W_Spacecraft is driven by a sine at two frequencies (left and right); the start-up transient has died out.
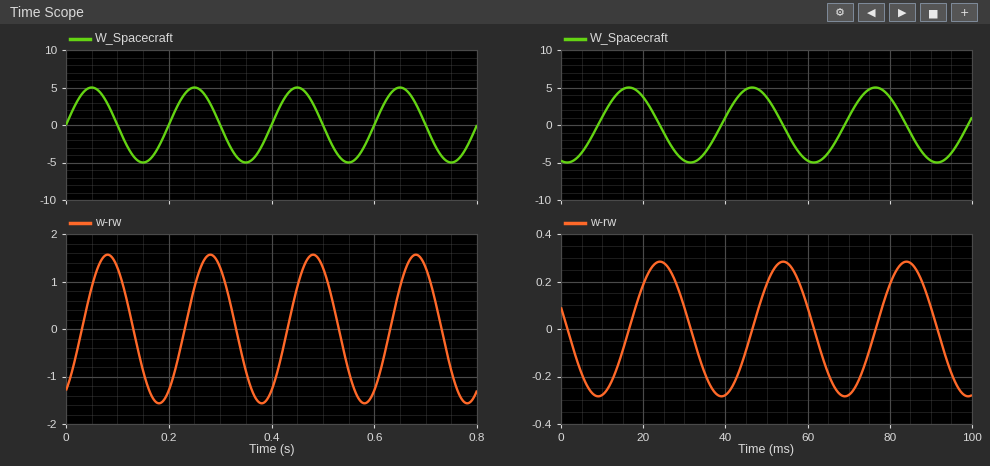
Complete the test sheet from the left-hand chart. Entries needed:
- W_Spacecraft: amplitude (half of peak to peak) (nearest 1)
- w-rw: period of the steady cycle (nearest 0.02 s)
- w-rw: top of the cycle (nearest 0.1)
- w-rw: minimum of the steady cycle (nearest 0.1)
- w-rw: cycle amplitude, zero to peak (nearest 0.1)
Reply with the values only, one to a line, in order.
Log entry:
5
0.20 s
1.6
-1.6
1.6
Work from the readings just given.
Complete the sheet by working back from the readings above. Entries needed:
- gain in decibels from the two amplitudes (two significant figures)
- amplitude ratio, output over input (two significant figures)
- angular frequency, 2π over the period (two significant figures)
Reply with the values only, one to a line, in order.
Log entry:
-9.9 dB
0.32
31 rad/s
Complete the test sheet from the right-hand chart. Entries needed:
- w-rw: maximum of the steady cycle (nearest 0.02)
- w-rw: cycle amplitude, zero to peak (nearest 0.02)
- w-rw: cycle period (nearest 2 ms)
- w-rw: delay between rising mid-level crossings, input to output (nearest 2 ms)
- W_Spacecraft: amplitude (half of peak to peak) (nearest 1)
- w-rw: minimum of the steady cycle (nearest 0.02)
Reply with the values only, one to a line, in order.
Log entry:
0.28
0.28
30 ms
8 ms
5
-0.28
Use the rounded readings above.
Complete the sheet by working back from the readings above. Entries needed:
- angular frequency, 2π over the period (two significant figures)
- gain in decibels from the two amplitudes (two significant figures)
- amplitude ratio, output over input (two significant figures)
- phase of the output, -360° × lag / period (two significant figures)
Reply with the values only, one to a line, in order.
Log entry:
0.21 rad/ms
-25 dB
0.056
-96°
